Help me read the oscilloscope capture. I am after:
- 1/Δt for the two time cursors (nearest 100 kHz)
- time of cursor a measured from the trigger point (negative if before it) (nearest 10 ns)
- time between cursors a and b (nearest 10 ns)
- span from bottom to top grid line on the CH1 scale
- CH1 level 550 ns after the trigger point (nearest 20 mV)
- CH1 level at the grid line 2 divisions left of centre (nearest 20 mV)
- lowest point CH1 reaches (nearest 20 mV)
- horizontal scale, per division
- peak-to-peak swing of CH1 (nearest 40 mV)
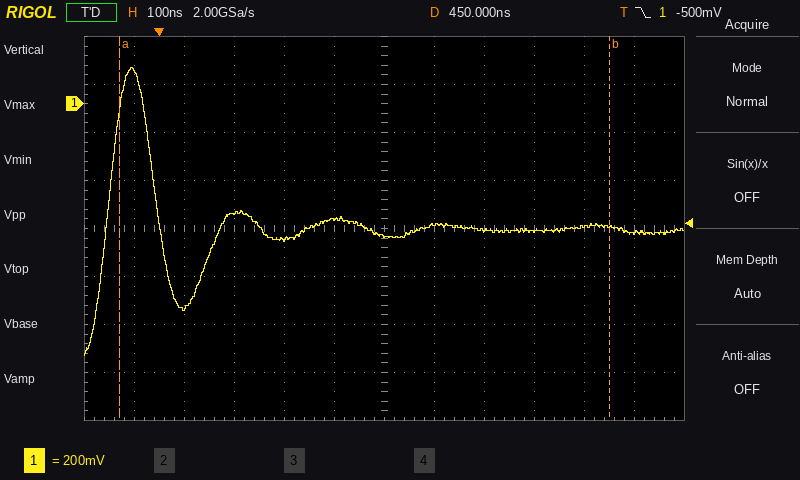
1.0 MHz
-80 ns
980 ns
1.6 V
-500 mV
-560 mV
-1.04 V
100 ns
1.20 V
